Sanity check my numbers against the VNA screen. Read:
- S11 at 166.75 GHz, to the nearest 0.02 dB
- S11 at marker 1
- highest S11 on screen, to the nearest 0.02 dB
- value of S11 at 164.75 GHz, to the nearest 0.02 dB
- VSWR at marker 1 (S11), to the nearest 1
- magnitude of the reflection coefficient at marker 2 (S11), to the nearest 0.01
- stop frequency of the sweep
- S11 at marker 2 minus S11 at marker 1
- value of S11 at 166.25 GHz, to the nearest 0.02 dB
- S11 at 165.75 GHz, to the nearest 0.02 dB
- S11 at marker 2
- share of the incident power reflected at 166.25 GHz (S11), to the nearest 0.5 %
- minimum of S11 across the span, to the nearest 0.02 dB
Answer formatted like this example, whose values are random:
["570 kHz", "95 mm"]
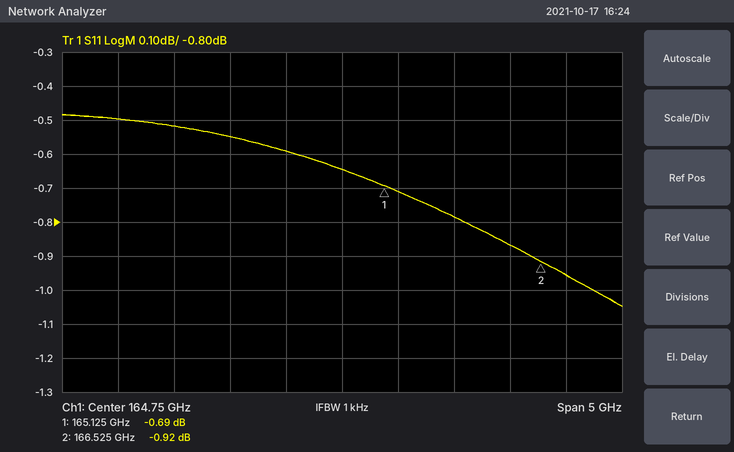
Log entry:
["-0.96 dB", "-0.69 dB", "-0.48 dB", "-0.64 dB", "25", "0.90", "167.25 GHz", "-0.23 dB", "-0.86 dB", "-0.78 dB", "-0.92 dB", "82.0 %", "-1.04 dB"]
